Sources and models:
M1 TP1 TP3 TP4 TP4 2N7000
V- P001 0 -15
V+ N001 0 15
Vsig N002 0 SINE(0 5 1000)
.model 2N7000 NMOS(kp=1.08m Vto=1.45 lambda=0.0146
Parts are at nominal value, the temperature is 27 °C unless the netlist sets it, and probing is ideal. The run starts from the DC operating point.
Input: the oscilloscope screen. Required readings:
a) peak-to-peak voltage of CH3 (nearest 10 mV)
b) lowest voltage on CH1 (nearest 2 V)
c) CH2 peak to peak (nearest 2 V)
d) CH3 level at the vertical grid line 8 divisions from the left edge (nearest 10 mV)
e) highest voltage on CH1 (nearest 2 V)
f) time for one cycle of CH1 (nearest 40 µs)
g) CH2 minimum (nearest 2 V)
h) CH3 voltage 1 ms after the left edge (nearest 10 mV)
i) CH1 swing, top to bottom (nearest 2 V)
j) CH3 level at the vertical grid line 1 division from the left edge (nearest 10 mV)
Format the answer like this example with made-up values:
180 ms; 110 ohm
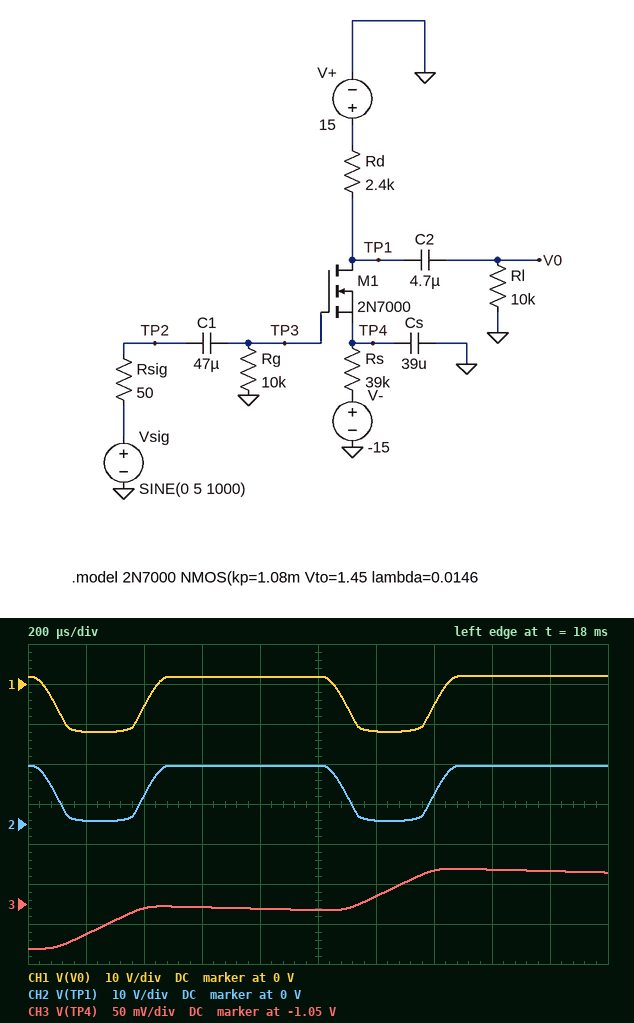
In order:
100 mV; -12 V; 14 V; -1.01 V; 2 V; 1.00 ms; 0 V; -1.06 V; 14 V; -1.09 V
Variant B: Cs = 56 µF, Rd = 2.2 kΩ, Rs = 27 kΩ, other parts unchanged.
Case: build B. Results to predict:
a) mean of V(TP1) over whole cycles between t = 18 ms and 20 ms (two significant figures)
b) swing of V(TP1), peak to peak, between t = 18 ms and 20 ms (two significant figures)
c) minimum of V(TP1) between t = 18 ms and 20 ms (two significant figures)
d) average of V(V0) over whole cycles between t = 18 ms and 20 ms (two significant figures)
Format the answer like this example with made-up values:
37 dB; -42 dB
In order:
9.8 V; 14 V; 250 mV; -2.6 V
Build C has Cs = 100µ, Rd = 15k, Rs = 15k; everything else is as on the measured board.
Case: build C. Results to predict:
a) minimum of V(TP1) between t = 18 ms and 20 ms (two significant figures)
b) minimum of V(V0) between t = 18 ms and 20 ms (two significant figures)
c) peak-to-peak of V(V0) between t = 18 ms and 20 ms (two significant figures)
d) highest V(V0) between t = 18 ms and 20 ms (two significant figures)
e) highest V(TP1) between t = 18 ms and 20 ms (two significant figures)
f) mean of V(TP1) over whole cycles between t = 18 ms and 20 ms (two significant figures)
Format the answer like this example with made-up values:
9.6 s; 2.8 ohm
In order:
-2.4 V; -5.0 V; 10 V; 5.0 V; 7.6 V; 2.6 V
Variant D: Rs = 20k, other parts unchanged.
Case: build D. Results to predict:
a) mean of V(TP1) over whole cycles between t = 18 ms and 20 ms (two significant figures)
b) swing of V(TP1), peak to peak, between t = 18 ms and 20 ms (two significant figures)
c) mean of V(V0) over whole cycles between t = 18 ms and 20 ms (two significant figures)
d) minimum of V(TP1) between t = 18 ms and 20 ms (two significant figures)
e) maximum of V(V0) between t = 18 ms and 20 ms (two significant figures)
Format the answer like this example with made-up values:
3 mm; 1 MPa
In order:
9.7 V; 14 V; -2.3 V; 210 mV; 2.4 V
